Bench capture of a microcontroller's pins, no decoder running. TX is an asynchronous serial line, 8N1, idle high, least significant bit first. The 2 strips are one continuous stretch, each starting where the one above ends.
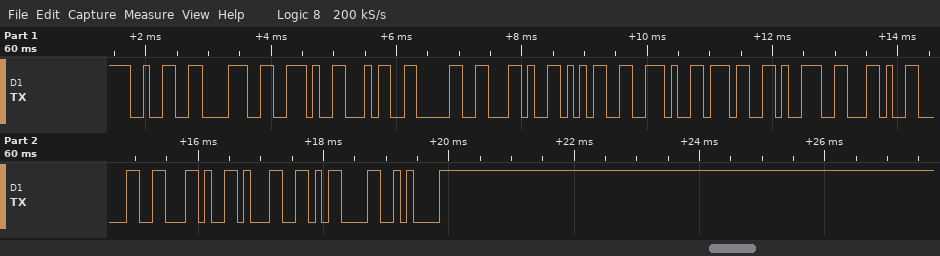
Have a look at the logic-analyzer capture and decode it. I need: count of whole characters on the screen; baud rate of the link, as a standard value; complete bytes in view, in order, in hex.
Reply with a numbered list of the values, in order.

1. 16
2. 9600 baud
3. 0x32 0x38 0x2E 0x34 0x30 0x2C 0x35 0x2E 0x37 0x39 0x2C 0x30 0x2C 0x31 0x0D 0x0A
